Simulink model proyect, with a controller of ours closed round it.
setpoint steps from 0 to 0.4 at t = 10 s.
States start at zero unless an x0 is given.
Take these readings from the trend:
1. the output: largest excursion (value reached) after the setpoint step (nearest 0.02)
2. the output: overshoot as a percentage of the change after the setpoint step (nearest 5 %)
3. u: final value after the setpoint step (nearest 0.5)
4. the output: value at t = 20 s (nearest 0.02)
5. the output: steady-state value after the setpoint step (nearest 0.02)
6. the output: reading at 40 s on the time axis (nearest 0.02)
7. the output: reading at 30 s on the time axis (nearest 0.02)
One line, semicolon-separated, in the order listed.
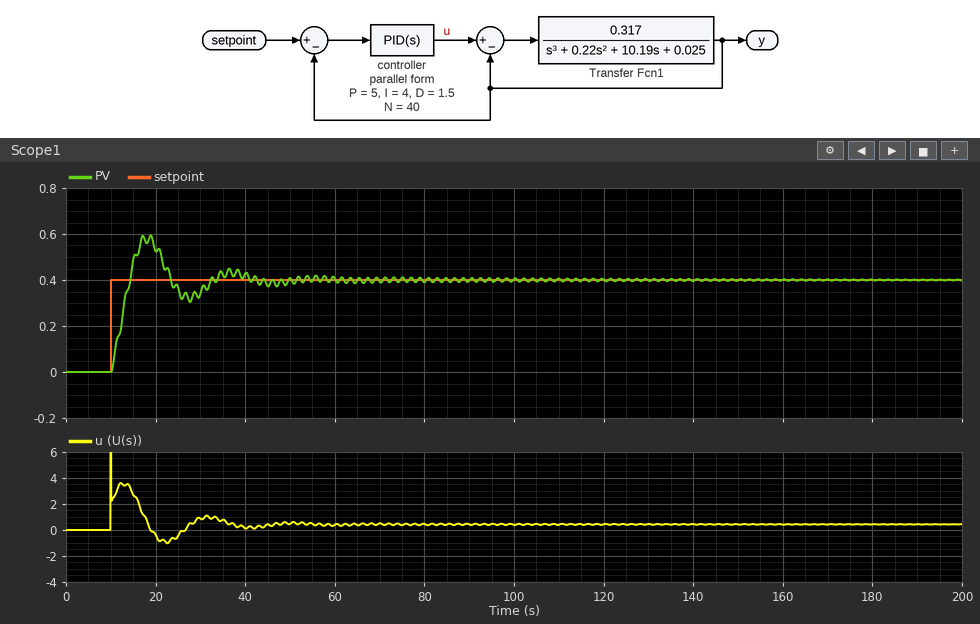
0.60; 50 %; 0.5; 0.52; 0.40; 0.42; 0.34
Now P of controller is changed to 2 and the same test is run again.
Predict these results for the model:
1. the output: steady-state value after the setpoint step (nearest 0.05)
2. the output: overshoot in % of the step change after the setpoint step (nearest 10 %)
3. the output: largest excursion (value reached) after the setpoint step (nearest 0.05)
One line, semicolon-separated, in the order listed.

0.40; 70 %; 0.65
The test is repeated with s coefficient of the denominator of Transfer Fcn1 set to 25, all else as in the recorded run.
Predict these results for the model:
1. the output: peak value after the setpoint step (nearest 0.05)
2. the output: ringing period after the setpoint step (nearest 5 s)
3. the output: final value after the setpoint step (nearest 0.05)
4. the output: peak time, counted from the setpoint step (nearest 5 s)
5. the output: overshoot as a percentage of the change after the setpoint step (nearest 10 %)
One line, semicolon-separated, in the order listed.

0.65; 30 s; 0.40; 15 s; 60 %
